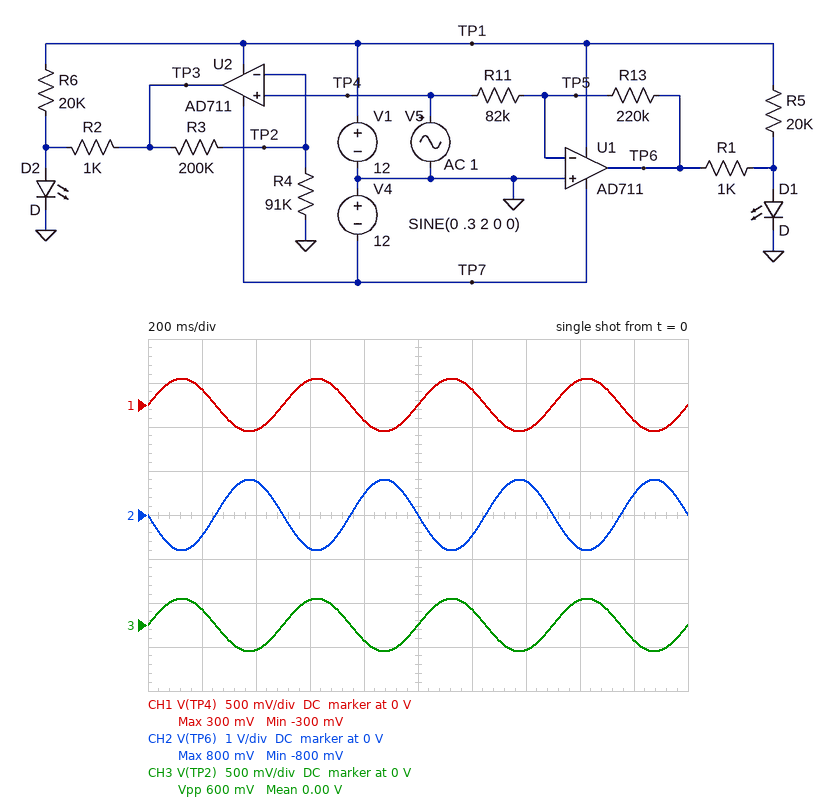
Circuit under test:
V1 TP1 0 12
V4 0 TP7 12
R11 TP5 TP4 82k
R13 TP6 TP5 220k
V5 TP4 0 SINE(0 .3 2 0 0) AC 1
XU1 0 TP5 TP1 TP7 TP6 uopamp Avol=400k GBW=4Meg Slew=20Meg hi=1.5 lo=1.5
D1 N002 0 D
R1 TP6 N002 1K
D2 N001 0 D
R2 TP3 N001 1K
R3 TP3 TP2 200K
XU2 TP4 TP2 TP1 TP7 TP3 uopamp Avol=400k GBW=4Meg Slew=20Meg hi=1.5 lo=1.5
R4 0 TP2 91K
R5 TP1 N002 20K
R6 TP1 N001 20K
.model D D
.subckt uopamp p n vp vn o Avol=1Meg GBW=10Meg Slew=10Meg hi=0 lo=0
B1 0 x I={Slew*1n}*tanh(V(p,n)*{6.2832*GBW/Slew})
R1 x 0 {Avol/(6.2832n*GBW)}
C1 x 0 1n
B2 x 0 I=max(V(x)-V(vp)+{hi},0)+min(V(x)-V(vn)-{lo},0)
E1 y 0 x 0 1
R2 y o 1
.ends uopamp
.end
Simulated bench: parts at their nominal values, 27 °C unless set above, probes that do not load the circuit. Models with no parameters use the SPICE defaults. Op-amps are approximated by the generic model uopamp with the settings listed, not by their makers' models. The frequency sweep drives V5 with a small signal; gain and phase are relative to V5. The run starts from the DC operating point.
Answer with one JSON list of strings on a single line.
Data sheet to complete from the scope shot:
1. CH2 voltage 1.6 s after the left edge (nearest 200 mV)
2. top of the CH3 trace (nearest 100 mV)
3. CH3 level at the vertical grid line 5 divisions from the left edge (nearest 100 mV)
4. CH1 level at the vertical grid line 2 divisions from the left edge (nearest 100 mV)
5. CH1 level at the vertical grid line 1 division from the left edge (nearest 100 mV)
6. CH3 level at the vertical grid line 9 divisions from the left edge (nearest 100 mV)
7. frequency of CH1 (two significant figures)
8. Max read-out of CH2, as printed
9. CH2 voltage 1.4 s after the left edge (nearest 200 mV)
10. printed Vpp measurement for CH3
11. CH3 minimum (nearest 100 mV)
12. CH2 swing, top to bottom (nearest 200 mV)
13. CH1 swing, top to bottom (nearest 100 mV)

["-800 mV", "300 mV", "0 V", "-300 mV", "200 mV", "-200 mV", "2.0 Hz", "800 mV", "800 mV", "600 mV", "-300 mV", "1.6 V", "600 mV"]
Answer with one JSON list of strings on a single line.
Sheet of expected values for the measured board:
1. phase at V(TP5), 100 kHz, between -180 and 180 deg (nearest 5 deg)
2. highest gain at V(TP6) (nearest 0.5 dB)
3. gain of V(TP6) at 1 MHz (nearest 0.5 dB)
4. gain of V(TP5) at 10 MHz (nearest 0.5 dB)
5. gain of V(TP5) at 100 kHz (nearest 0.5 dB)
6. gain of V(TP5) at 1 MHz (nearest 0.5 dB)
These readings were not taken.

["85 deg", "8.5 dB", "6.0 dB", "-3.0 dB", "-23.5 dB", "-6.0 dB"]
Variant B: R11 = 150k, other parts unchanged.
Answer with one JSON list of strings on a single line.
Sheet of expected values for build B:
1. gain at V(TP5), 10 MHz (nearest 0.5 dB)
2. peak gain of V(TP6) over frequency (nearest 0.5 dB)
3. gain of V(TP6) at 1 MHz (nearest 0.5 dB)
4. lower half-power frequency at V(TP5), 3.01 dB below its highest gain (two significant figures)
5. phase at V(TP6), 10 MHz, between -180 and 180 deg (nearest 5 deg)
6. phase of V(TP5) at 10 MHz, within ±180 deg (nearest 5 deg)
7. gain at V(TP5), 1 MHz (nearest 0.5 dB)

["-4.5 dB", "3.5 dB", "2.0 dB", "1.6 MHz", "100 deg", "10 deg", "-10.0 dB"]
